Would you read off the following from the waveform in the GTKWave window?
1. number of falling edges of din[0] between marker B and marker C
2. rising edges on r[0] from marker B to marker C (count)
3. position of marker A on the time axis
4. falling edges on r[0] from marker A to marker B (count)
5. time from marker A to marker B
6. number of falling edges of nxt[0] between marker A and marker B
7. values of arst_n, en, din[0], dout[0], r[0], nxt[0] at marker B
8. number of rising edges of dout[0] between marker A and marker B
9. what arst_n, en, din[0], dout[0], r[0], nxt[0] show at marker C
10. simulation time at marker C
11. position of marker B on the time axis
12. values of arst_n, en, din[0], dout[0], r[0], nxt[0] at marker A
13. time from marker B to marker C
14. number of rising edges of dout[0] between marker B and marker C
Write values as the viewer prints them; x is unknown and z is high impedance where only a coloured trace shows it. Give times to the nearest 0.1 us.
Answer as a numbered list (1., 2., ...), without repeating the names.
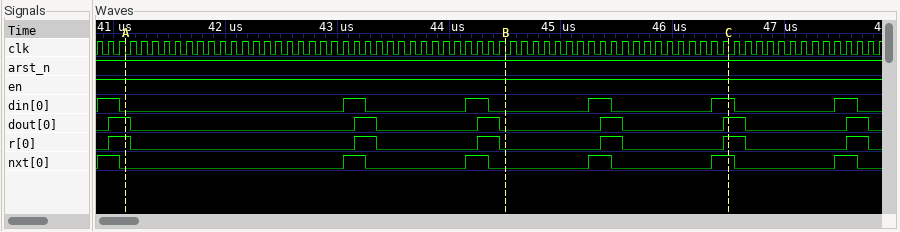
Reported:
1. 1
2. 2
3. 41.1 us
4. 3
5. 3.4 us
6. 2
7. arst_n=1, en=1, din[0]=0, dout[0]=0, r[0]=0, nxt[0]=0
8. 2
9. arst_n=1, en=1, din[0]=1, dout[0]=1, r[0]=1, nxt[0]=1
10. 46.5 us
11. 44.5 us
12. arst_n=1, en=1, din[0]=0, dout[0]=1, r[0]=1, nxt[0]=0
13. 2 us
14. 2
